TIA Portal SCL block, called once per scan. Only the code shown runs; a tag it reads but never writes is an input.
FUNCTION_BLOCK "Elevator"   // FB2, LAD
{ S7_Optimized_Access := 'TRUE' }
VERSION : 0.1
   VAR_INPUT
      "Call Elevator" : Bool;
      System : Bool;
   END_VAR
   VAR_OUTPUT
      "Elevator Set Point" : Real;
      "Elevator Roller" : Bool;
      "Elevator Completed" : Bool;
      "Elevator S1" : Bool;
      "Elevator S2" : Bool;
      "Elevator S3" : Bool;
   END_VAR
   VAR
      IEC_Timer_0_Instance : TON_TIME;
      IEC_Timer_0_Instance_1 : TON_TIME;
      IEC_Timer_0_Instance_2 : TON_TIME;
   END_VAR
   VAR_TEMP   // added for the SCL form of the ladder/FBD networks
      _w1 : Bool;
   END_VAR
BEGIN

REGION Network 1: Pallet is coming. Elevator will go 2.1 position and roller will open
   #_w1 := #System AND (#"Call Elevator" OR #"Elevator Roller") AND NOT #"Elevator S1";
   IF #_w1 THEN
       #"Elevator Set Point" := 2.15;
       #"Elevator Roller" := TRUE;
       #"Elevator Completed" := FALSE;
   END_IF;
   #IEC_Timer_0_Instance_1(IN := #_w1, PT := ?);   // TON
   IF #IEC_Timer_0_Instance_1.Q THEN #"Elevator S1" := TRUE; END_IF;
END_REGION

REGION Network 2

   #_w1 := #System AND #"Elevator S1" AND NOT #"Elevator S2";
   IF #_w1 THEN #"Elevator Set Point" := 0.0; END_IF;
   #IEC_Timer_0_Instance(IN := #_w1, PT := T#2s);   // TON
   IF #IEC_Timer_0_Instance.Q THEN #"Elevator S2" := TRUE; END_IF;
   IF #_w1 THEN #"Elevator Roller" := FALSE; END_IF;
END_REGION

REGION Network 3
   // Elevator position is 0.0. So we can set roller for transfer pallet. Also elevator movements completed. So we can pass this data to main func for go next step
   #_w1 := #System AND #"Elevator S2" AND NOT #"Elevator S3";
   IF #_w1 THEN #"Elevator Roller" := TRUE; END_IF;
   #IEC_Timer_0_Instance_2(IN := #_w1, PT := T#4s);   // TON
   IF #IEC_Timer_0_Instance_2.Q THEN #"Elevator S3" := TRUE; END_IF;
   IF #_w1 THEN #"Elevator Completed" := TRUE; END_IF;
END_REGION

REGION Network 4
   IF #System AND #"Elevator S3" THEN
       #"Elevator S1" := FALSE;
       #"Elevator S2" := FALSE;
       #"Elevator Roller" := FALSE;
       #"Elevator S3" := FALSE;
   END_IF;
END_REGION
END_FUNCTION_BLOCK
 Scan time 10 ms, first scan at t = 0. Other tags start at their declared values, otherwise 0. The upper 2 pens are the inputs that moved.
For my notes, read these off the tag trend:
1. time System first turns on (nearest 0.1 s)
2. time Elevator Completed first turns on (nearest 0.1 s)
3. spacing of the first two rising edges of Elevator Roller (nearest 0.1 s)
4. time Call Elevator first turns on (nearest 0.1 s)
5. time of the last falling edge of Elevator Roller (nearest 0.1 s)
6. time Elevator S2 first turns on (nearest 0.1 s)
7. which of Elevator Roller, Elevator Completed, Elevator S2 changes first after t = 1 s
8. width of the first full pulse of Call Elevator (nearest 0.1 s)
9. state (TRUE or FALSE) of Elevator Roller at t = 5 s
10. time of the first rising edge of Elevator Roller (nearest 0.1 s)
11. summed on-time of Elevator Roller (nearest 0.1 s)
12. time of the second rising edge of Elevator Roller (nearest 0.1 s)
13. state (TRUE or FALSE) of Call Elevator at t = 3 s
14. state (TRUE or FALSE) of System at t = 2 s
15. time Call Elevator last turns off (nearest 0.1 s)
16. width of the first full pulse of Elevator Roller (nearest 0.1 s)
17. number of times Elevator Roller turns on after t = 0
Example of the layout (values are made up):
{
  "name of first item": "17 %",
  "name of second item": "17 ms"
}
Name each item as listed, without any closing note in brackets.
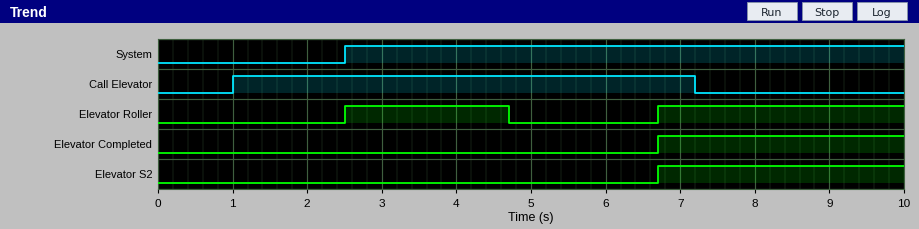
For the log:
{
  "time System first turns on": "2.5 s",
  "time Elevator Completed first turns on": "6.7 s",
  "spacing of the first two rising edges of Elevator Roller": "4.2 s",
  "time Call Elevator first turns on": "1.0 s",
  "time of the last falling edge of Elevator Roller": "4.7 s",
  "time Elevator S2 first turns on": "6.7 s",
  "which of Elevator Roller, Elevator Completed, Elevator S2 changes first after t = 1 s": "Elevator Roller",
  "width of the first full pulse of Call Elevator": "6.2 s",
  "state (TRUE or FALSE) of Elevator Roller at t = 5 s": "FALSE",
  "time of the first rising edge of Elevator Roller": "2.5 s",
  "summed on-time of Elevator Roller": "5.5 s",
  "time of the second rising edge of Elevator Roller": "6.7 s",
  "state (TRUE or FALSE) of Call Elevator at t = 3 s": "TRUE",
  "state (TRUE or FALSE) of System at t = 2 s": "FALSE",
  "time Call Elevator last turns off": "7.2 s",
  "width of the first full pulse of Elevator Roller": "2.2 s",
  "number of times Elevator Roller turns on after t = 0": "2"
}
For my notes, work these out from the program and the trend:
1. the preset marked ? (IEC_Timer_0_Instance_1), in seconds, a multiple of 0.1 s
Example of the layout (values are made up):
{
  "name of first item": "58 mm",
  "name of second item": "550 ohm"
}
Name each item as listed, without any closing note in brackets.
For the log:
{
  "the preset marked ? (IEC_Timer_0_Instance_1), in seconds, a multiple of 0.1 s": "2.2 s"
}
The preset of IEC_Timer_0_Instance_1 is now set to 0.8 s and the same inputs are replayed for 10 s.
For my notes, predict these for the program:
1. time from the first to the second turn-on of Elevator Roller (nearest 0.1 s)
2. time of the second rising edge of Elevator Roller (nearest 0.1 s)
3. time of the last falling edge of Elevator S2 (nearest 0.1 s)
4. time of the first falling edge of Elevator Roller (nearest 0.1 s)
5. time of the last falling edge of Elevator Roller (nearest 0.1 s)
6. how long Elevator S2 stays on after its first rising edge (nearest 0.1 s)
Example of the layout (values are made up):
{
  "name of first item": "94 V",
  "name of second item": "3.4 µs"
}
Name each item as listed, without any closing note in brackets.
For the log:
{
  "time from the first to the second turn-on of Elevator Roller": "2.8 s",
  "time of the second rising edge of Elevator Roller": "5.3 s",
  "time of the last falling edge of Elevator S2": "9.3 s",
  "time of the first falling edge of Elevator Roller": "3.3 s",
  "time of the last falling edge of Elevator Roller": "9.3 s",
  "how long Elevator S2 stays on after its first rising edge": "4.0 s"
}
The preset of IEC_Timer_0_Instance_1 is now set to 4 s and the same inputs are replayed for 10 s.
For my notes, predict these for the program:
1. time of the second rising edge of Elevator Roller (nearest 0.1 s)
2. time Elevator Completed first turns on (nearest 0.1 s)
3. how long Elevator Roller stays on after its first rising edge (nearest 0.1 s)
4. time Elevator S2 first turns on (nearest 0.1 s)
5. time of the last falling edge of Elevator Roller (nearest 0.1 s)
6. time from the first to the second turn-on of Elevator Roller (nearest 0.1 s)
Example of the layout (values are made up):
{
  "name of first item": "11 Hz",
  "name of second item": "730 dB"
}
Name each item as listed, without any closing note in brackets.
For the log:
{
  "time of the second rising edge of Elevator Roller": "8.5 s",
  "time Elevator Completed first turns on": "8.5 s",
  "how long Elevator Roller stays on after its first rising edge": "4.0 s",
  "time Elevator S2 first turns on": "8.5 s",
  "time of the last falling edge of Elevator Roller": "6.5 s",
  "time from the first to the second turn-on of Elevator Roller": "6.0 s"
}
